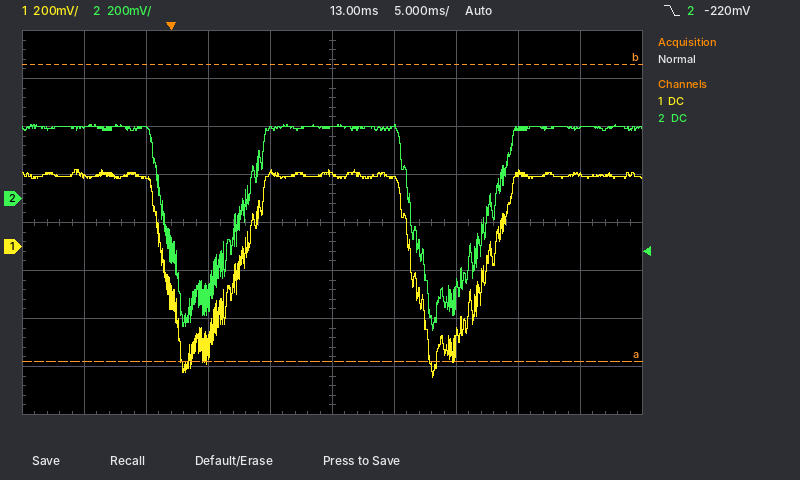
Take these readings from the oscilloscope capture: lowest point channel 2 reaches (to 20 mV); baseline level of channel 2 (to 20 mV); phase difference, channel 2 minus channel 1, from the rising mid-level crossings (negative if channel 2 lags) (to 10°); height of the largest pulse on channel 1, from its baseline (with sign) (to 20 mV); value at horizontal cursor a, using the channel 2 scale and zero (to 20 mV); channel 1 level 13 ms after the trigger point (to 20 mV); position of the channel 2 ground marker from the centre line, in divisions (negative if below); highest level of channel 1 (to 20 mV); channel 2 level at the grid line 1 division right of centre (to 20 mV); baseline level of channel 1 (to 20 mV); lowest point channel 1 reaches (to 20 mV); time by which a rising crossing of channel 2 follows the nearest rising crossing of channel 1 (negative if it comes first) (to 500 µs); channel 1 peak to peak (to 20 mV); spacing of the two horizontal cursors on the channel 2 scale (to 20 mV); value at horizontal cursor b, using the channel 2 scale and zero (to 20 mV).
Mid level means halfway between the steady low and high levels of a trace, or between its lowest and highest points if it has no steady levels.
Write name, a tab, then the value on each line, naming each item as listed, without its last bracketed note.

lowest point channel 2 reaches	-560 mV
baseline level of channel 2	300 mV
phase difference, channel 2 minus channel 1, from the rising mid-level crossings (negative if channel 2 lags)	0°
height of the largest pulse on channel 1, from its baseline (with sign)	-840 mV
value at horizontal cursor a, using the channel 2 scale and zero	-680 mV
channel 1 level 13 ms after the trigger point	300 mV
position of the channel 2 ground marker from the centre line, in divisions	+0.5 div
highest level of channel 1	320 mV
channel 2 level at the grid line 1 division right of centre	300 mV
baseline level of channel 1	300 mV
lowest point channel 1 reaches	-540 mV
time by which a rising crossing of channel 2 follows the nearest rising crossing of channel 1 (negative if it comes first)	0.0 ms
channel 1 peak to peak	860 mV
spacing of the two horizontal cursors on the channel 2 scale	1.24 V
value at horizontal cursor b, using the channel 2 scale and zero	560 mV
